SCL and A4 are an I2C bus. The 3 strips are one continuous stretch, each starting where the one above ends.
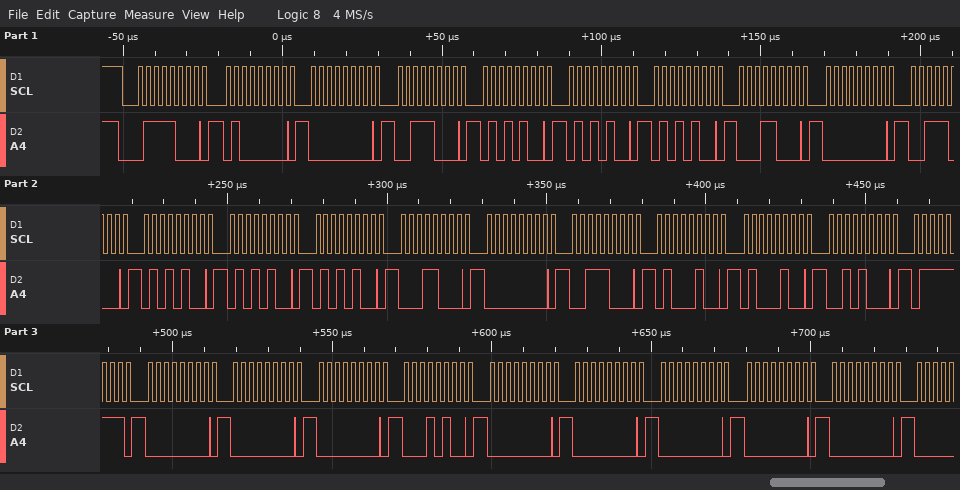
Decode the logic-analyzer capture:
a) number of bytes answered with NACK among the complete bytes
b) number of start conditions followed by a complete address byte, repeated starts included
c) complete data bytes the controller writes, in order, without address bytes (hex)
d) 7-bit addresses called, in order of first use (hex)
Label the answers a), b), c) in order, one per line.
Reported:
a) 0
b) 1
c) 40 00 38 54 54 54 18 00 38 54 54 54 18 00 38 44 44 28 7F 00 00 00 14 00 00 00 00 00
d) 0x3C
